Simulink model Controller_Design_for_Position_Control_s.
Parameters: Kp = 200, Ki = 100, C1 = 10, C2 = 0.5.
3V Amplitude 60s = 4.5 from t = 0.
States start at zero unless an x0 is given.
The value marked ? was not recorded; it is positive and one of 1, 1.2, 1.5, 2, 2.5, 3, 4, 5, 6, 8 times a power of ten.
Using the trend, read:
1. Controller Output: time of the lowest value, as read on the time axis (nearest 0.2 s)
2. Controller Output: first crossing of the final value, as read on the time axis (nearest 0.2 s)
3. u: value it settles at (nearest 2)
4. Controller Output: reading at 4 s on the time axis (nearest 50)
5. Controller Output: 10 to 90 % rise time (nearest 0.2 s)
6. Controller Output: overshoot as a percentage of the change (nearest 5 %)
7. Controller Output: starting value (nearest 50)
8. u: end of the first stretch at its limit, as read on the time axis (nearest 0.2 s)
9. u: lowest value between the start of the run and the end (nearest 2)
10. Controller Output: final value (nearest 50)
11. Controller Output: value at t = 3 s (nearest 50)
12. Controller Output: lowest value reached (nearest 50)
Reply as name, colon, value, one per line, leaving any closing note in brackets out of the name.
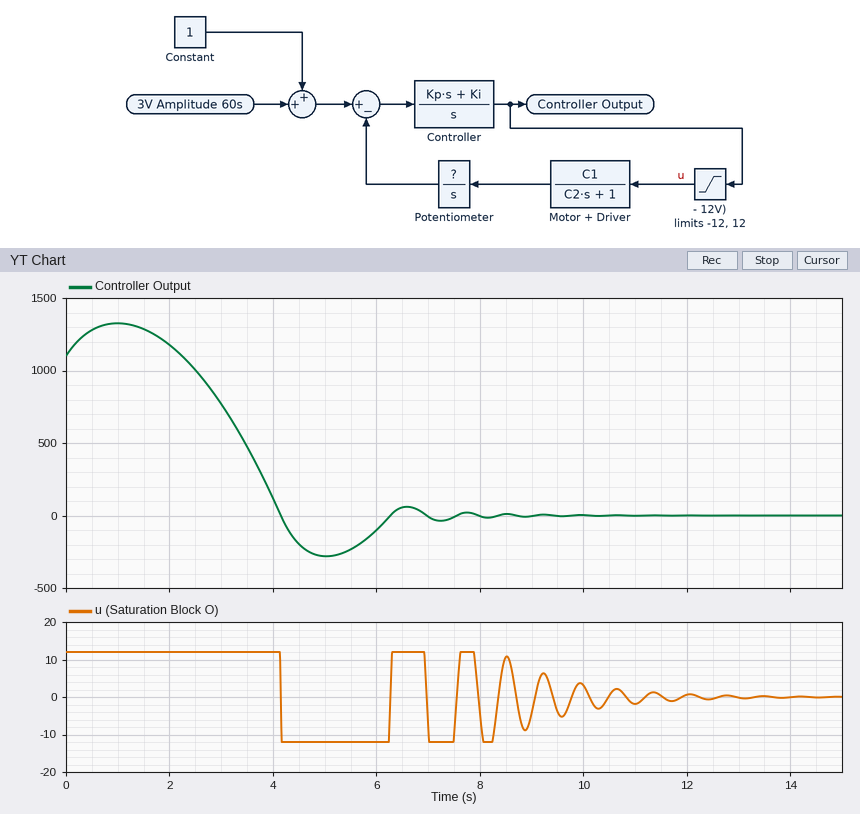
Controller Output: time of the lowest value, as read on the time axis: 5.0 s
Controller Output: first crossing of the final value, as read on the time axis: 4.2 s
u: value it settles at: 0
Controller Output: reading at 4 s on the time axis: 100
Controller Output: 10 to 90 % rise time: 1.4 s
Controller Output: overshoot as a percentage of the change: 25 %
Controller Output: starting value: 1100
u: end of the first stretch at its limit, as read on the time axis: 4.2 s
u: lowest value between the start of the run and the end: -12
Controller Output: final value: 0
Controller Output: value at t = 3 s: 750
Controller Output: lowest value reached: -300
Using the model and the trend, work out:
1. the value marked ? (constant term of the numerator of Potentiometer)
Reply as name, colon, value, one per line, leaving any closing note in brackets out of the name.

the value marked ?: 0.02
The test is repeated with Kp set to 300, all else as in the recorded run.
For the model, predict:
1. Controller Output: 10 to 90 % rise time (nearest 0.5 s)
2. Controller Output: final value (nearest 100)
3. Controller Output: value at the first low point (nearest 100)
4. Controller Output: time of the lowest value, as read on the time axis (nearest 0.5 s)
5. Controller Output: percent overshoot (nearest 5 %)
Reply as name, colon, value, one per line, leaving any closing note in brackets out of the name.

Controller Output: 10 to 90 % rise time: 2.0 s
Controller Output: final value: 0
Controller Output: value at the first low point: -200
Controller Output: time of the lowest value, as read on the time axis: 4.5 s
Controller Output: percent overshoot: 15 %
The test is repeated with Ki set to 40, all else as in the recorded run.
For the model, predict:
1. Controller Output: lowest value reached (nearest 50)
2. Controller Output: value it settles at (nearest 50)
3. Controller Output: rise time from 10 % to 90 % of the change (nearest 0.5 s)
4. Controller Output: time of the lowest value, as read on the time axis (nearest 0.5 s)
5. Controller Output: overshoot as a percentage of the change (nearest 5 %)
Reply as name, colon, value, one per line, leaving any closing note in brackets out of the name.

Controller Output: lowest value reached: -100
Controller Output: value it settles at: 0
Controller Output: rise time from 10 % to 90 % of the change: 2.0 s
Controller Output: time of the lowest value, as read on the time axis: 4.0 s
Controller Output: overshoot as a percentage of the change: 10 %
